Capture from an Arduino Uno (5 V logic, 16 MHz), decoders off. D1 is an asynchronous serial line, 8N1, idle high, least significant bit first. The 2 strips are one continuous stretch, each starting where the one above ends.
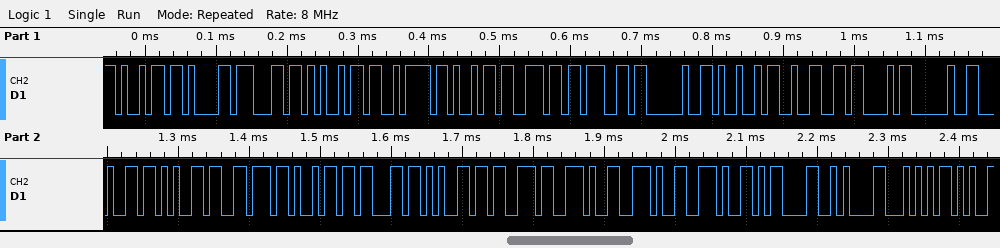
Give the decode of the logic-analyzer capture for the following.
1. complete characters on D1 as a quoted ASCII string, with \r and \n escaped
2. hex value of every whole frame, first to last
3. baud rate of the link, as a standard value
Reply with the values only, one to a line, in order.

"ializing I2C devices...\r\nT"
69 61 6C 69 7A 69 6E 67 20 49 32 43 20 64 65 76 69 63 65 73 2E 2E 2E 0D 0A 54
115200 baud
